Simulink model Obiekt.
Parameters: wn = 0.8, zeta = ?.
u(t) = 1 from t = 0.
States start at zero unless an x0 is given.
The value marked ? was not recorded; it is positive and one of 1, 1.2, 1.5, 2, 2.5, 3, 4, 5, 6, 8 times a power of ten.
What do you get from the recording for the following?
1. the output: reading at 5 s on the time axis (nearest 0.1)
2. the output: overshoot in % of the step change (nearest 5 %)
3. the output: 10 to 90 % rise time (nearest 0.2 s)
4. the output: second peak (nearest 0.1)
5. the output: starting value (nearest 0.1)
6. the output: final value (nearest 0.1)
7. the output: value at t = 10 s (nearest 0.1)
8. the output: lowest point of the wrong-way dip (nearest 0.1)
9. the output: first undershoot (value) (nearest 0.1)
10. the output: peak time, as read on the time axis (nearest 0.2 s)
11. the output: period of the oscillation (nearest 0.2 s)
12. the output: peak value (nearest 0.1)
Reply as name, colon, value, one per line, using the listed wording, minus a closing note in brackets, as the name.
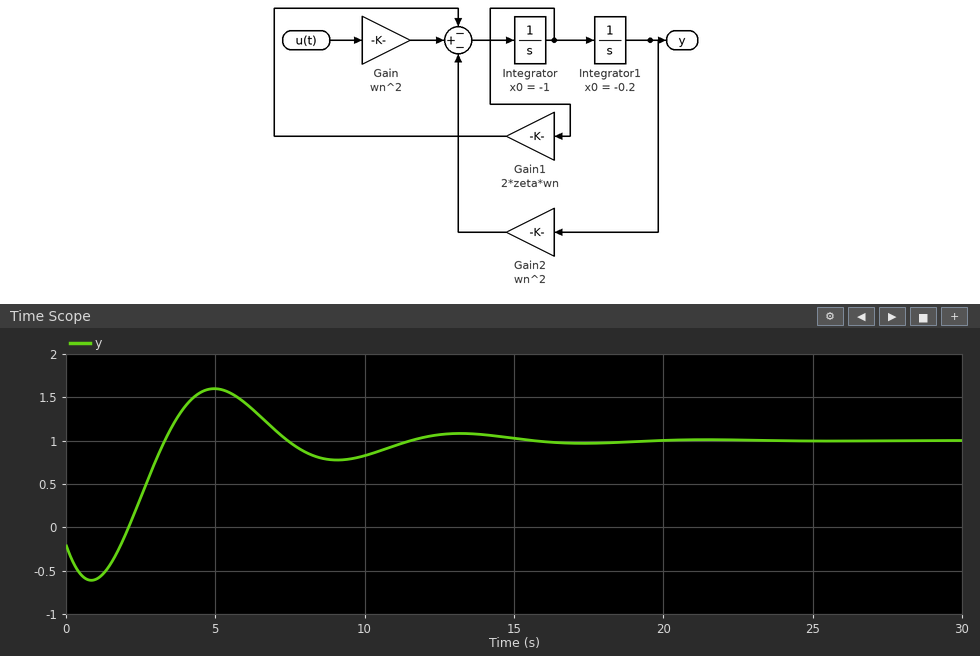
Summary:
the output: reading at 5 s on the time axis: 1.6
the output: overshoot in % of the step change: 50 %
the output: 10 to 90 % rise time: 1.2 s
the output: second peak: 1.1
the output: starting value: -0.2
the output: final value: 1.0
the output: value at t = 10 s: 0.8
the output: lowest point of the wrong-way dip: -0.6
the output: first undershoot (value): 0.8
the output: peak time, as read on the time axis: 5.0 s
the output: period of the oscillation: 8.2 s
the output: peak value: 1.6
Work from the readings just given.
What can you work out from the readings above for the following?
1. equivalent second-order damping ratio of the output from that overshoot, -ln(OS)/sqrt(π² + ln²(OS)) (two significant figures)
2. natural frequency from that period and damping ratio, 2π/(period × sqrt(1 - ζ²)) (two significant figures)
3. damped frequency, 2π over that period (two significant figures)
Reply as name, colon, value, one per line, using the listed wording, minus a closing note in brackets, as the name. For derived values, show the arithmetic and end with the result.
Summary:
equivalent second-order damping ratio of the output from that overshoot, -ln(OS)/sqrt(π² + ln²(OS)): ln(0.5) = -0.693; 0.693 / sqrt(9.870 + 0.480) = 0.22
natural frequency from that period and damping ratio, 2π/(period × sqrt(1 - ζ²)): 2π / (8.2 × sqrt(1 - 0.22²)) = 0.79 rad/s
damped frequency, 2π over that period: 2π / 8.2 = 0.77 rad/s
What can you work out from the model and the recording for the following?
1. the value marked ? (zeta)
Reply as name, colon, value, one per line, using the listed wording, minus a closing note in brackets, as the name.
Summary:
the value marked ?: 0.3
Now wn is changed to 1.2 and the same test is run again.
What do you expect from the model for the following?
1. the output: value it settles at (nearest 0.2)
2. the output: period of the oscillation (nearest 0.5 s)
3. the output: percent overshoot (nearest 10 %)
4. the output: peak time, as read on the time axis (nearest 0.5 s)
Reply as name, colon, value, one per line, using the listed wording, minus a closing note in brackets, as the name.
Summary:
the output: value it settles at: 1.0
the output: period of the oscillation: 5.5 s
the output: percent overshoot: 40 %
the output: peak time, as read on the time axis: 3.0 s
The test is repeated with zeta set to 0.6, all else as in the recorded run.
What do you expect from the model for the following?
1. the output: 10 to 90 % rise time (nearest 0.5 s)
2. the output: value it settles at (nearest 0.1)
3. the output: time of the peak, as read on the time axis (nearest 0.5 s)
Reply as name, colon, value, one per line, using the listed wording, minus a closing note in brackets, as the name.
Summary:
the output: 10 to 90 % rise time: 2.0 s
the output: value it settles at: 1.0
the output: time of the peak, as read on the time axis: 5.5 s
